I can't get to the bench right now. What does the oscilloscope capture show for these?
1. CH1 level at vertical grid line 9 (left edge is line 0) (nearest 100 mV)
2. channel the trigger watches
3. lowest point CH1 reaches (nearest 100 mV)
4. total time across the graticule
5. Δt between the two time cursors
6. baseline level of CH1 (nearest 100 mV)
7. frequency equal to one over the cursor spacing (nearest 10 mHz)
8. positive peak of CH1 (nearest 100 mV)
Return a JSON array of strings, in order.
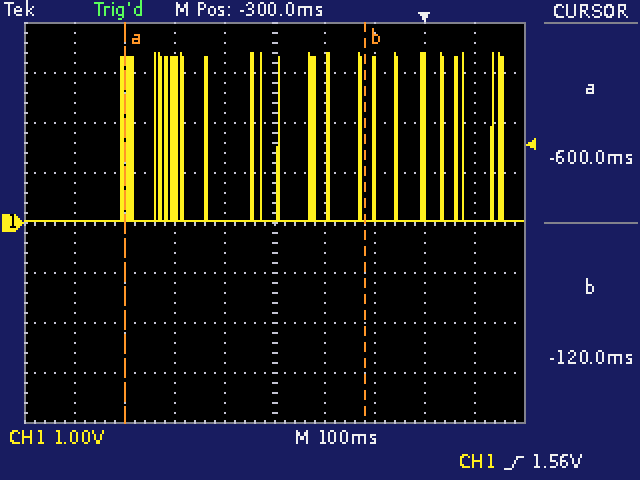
["0.0 V", "CH1", "0.0 V", "1 s", "480 ms", "0.0 V", "2.08 Hz", "3.4 V"]
